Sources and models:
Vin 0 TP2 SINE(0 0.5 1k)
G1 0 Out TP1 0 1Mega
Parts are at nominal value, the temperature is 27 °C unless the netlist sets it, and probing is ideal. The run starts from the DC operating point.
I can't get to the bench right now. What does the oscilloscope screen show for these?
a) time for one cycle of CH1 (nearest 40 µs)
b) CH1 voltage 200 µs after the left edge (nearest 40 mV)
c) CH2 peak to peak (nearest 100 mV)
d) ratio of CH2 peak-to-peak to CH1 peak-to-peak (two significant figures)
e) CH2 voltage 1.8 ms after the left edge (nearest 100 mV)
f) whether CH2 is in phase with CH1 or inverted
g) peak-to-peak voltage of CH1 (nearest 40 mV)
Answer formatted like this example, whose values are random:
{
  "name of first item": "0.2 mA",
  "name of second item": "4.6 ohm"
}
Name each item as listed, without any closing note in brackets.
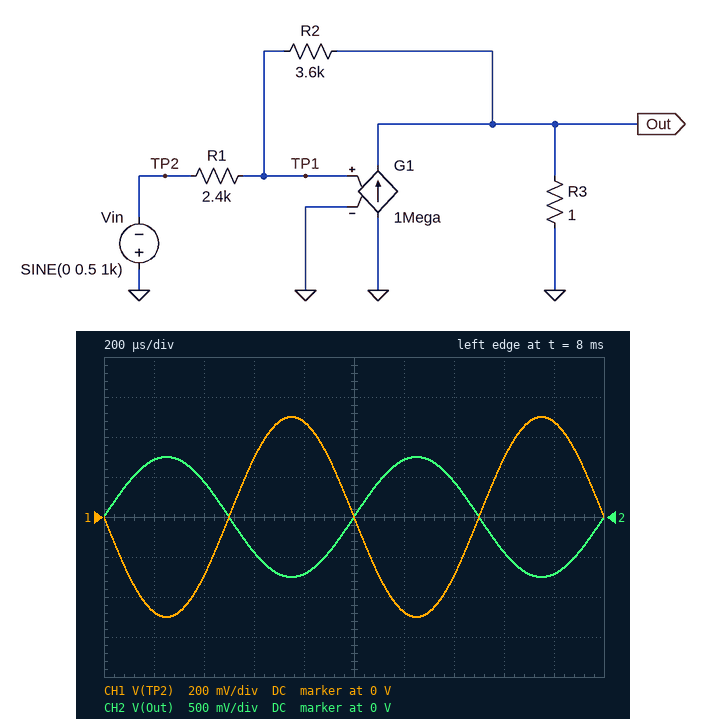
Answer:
{
  "time for one cycle of CH1": "1.00 ms",
  "CH1 voltage 200 µs after the left edge": "-480 mV",
  "CH2 peak to peak": "1.5 V",
  "ratio of CH2 peak-to-peak to CH1 peak-to-peak": "1.5",
  "CH2 voltage 1.8 ms after the left edge": "-700 mV",
  "whether CH2 is in phase with CH1 or inverted": "inverted",
  "peak-to-peak voltage of CH1": "1.00 V"
}
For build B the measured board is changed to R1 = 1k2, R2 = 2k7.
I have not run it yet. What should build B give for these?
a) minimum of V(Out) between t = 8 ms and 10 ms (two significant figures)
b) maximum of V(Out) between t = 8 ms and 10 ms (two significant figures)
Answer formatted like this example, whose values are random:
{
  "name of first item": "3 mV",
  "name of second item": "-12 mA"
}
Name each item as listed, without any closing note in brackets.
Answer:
{
  "minimum of V(Out) between t = 8 ms and 10 ms": "-1.1 V",
  "maximum of V(Out) between t = 8 ms and 10 ms": "1.1 V"
}
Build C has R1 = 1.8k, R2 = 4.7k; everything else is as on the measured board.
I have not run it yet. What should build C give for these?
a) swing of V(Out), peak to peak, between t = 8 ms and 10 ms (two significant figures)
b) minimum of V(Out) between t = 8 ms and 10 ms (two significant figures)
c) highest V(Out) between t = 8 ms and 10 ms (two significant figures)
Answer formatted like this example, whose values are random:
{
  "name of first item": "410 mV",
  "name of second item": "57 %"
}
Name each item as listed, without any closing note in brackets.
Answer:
{
  "swing of V(Out), peak to peak, between t = 8 ms and 10 ms": "2.6 V",
  "minimum of V(Out) between t = 8 ms and 10 ms": "-1.3 V",
  "highest V(Out) between t = 8 ms and 10 ms": "1.3 V"
}
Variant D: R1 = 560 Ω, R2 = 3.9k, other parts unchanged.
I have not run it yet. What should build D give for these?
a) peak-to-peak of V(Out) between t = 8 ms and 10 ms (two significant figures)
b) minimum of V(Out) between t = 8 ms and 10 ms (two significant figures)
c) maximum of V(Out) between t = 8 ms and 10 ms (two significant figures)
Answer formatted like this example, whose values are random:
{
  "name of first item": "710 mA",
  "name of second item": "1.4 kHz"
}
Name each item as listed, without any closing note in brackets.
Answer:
{
  "peak-to-peak of V(Out) between t = 8 ms and 10 ms": "7.0 V",
  "minimum of V(Out) between t = 8 ms and 10 ms": "-3.5 V",
  "maximum of V(Out) between t = 8 ms and 10 ms": "3.5 V"
}
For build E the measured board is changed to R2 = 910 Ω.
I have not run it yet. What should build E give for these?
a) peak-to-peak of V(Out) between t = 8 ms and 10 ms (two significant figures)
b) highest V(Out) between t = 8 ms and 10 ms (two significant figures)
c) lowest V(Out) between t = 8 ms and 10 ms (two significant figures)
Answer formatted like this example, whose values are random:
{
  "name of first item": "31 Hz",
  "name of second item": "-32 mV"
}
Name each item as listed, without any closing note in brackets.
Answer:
{
  "peak-to-peak of V(Out) between t = 8 ms and 10 ms": "380 mV",
  "highest V(Out) between t = 8 ms and 10 ms": "190 mV",
  "lowest V(Out) between t = 8 ms and 10 ms": "-190 mV"
}
